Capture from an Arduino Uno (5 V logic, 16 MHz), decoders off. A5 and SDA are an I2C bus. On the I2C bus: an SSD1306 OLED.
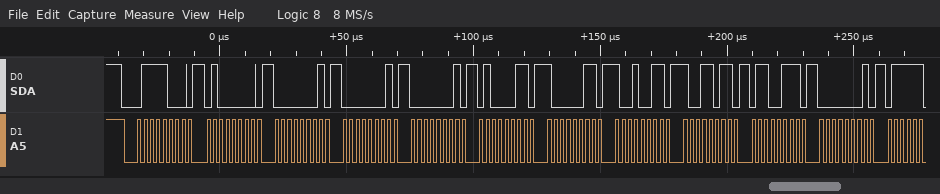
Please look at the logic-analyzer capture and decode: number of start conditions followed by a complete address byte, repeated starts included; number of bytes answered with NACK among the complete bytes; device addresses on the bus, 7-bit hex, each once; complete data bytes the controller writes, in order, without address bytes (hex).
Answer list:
1
0
0x3C
40 01 01 01 43 83 93 9B 67 01
